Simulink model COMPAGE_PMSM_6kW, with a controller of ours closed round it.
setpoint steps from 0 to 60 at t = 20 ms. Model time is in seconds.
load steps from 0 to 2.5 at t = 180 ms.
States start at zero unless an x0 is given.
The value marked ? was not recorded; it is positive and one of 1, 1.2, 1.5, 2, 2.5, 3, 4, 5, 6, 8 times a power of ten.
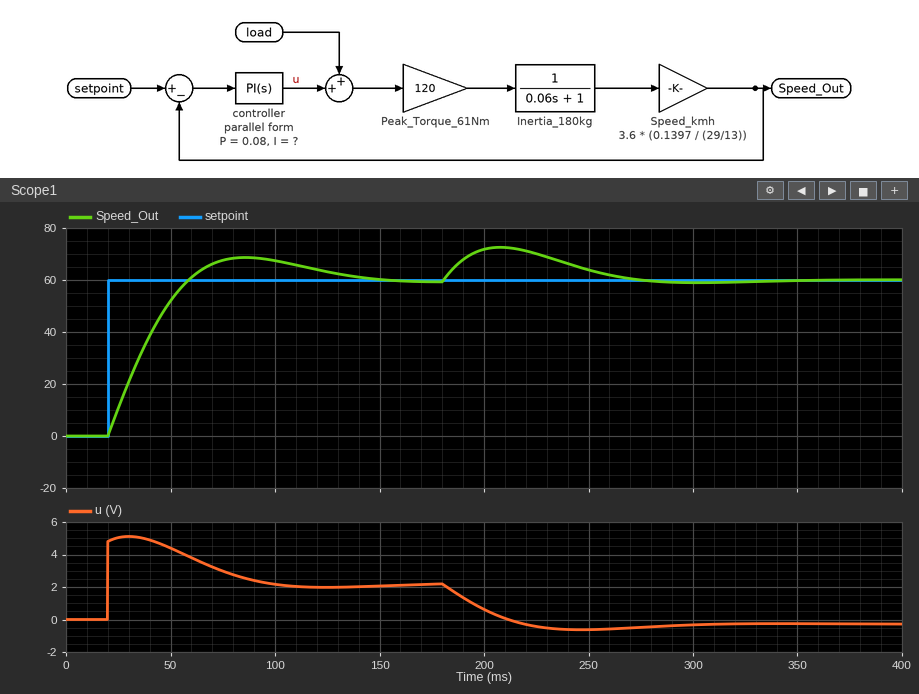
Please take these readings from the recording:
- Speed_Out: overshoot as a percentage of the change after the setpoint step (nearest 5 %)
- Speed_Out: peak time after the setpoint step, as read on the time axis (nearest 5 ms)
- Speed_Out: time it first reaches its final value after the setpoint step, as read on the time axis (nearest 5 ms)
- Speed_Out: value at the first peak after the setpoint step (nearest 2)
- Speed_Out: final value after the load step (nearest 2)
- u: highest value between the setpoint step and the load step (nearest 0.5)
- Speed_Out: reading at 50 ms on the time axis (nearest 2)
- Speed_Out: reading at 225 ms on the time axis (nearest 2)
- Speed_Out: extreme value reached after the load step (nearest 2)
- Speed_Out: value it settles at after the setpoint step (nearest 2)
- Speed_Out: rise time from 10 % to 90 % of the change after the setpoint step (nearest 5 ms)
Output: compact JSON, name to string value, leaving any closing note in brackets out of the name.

{"Speed_Out: overshoot as a percentage of the change after the setpoint step": "15 %", "Speed_Out: peak time after the setpoint step, as read on the time axis": "85 ms", "Speed_Out: time it first reaches its final value after the setpoint step, as read on the time axis": "60 ms", "Speed_Out: value at the first peak after the setpoint step": "68", "Speed_Out: final value after the load step": "60", "u: highest value between the setpoint step and the load step": "5.0", "Speed_Out: reading at 50 ms on the time axis": "52", "Speed_Out: reading at 225 ms on the time axis": "70", "Speed_Out: extreme value reached after the load step": "72", "Speed_Out: value it settles at after the setpoint step": "60", "Speed_Out: rise time from 10 % to 90 % of the change after the setpoint step": "30 ms"}
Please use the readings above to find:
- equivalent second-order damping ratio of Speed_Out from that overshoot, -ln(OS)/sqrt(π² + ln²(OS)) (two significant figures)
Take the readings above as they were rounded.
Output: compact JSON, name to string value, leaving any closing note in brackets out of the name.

{"equivalent second-order damping ratio of Speed_Out from that overshoot, -ln(OS)/sqrt(π² + ln²(OS))": "0.52"}
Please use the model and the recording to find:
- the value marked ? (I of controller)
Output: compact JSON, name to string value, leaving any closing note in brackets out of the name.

{"the value marked ?": "4"}
